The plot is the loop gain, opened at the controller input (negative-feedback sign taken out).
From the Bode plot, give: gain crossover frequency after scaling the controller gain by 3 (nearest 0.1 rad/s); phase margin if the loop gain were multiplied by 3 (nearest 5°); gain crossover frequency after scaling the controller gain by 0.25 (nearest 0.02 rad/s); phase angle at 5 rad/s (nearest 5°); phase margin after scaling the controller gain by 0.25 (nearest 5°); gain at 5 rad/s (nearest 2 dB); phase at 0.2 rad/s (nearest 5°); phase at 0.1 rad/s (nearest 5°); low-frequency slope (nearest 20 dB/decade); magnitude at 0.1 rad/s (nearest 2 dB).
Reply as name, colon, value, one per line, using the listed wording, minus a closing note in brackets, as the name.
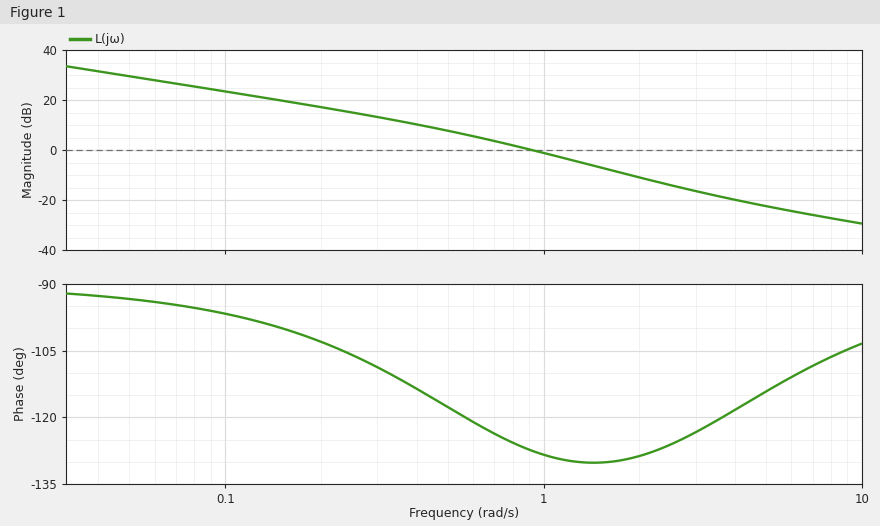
gain crossover frequency after scaling the controller gain by 3: 1.8 rad/s
phase margin if the loop gain were multiplied by 3: 50°
gain crossover frequency after scaling the controller gain by 0.25: 0.34 rad/s
phase angle at 5 rad/s: -115°
phase margin after scaling the controller gain by 0.25: 70°
gain at 5 rad/s: -22 dB
phase at 0.2 rad/s: -105°
phase at 0.1 rad/s: -95°
low-frequency slope: -20 dB/decade
magnitude at 0.1 rad/s: 24 dB
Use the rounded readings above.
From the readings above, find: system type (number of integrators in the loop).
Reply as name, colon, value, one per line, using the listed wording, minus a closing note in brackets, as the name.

system type: 1
